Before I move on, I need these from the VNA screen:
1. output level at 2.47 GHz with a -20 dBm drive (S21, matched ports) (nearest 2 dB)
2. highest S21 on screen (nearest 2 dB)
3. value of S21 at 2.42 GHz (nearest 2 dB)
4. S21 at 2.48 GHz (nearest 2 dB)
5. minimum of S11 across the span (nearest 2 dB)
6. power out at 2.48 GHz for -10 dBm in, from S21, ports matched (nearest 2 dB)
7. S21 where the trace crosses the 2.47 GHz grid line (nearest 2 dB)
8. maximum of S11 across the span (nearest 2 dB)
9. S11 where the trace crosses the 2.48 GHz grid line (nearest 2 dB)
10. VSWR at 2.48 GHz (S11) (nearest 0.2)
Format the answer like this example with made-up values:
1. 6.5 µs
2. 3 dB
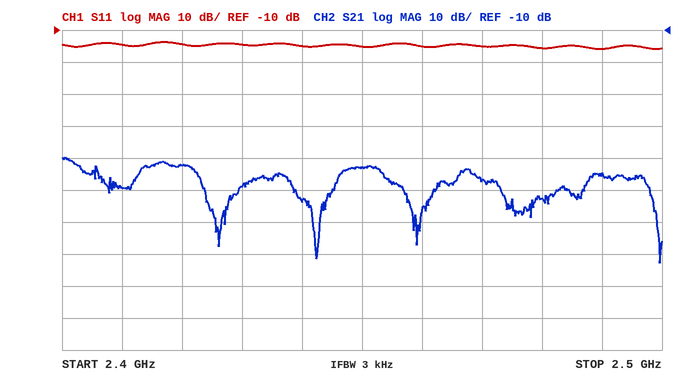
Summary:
1. -76 dBm
2. -50 dB
3. -52 dB
4. -62 dB
5. -16 dB
6. -72 dBm
7. -56 dB
8. -14 dB
9. -16 dB
10. 1.4
